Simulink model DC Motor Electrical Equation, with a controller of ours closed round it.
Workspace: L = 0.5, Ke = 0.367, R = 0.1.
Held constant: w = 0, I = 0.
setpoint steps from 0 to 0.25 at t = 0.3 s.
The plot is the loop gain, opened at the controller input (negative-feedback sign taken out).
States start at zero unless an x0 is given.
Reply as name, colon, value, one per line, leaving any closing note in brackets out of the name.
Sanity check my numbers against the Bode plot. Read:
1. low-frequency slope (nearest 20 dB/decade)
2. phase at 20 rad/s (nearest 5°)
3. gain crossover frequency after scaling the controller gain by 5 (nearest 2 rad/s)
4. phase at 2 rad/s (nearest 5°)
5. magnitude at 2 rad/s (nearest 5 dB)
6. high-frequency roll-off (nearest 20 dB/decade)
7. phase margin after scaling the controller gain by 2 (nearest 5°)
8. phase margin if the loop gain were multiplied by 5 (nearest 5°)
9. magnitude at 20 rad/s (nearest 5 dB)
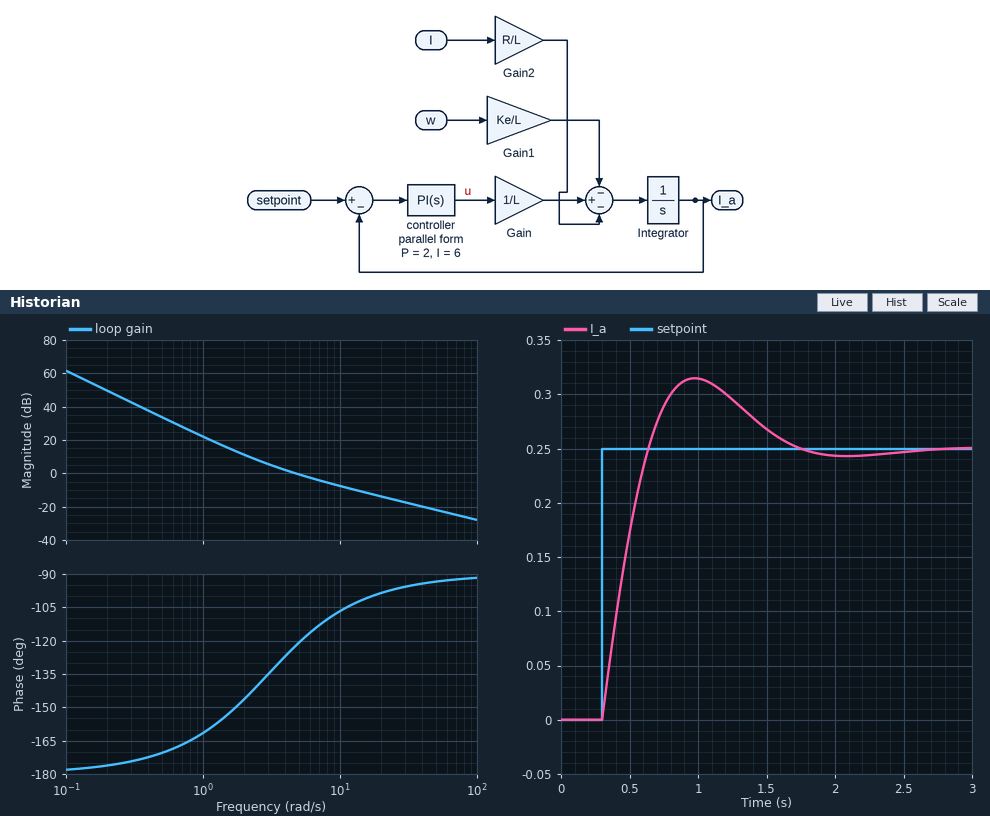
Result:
low-frequency slope: -40 dB/decade
phase at 20 rad/s: -100°
gain crossover frequency after scaling the controller gain by 5: 20 rad/s
phase at 2 rad/s: -145°
magnitude at 2 rad/s: 10 dB
high-frequency roll-off: -20 dB/decade
phase margin after scaling the controller gain by 2: 70°
phase margin if the loop gain were multiplied by 5: 80°
magnitude at 20 rad/s: -15 dB
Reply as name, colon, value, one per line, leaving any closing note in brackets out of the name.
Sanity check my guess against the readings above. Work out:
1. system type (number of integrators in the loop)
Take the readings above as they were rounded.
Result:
system type: 2
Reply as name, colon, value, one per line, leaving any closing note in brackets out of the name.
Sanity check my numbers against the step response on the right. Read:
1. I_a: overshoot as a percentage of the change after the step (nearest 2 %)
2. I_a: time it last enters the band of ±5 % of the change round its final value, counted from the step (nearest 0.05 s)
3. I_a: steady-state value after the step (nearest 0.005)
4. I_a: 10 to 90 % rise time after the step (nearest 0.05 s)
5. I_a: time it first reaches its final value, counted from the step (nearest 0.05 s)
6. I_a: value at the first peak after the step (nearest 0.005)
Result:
I_a: overshoot as a percentage of the change after the step: 26 %
I_a: time it last enters the band of ±5 % of the change round its final value, counted from the step: 1.25 s
I_a: steady-state value after the step: 0.250
I_a: 10 to 90 % rise time after the step: 0.25 s
I_a: time it first reaches its final value, counted from the step: 0.35 s
I_a: value at the first peak after the step: 0.315
